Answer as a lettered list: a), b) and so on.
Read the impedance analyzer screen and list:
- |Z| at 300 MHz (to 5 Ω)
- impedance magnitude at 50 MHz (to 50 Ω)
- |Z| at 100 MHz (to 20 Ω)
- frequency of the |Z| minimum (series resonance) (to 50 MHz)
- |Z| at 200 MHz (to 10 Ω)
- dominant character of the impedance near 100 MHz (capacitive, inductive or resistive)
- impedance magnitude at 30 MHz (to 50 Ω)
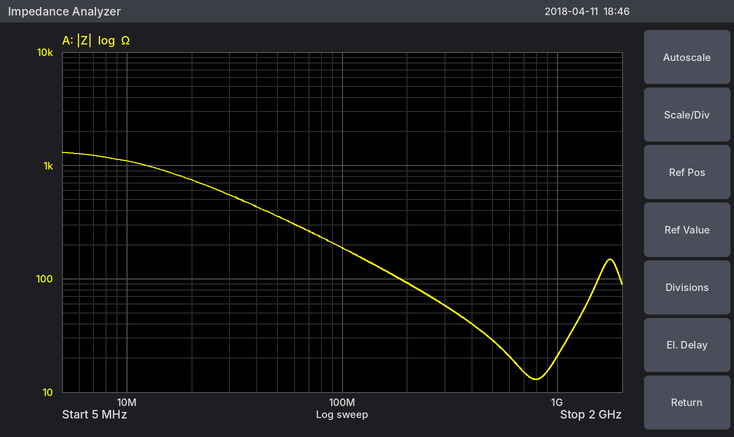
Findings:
a) 60 Ω
b) 350 Ω
c) 180 Ω
d) 800 MHz
e) 90 Ω
f) capacitive
g) 550 Ω
